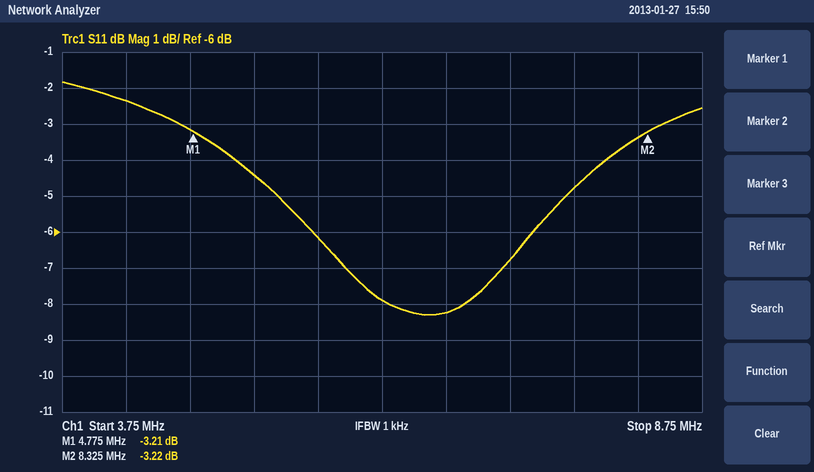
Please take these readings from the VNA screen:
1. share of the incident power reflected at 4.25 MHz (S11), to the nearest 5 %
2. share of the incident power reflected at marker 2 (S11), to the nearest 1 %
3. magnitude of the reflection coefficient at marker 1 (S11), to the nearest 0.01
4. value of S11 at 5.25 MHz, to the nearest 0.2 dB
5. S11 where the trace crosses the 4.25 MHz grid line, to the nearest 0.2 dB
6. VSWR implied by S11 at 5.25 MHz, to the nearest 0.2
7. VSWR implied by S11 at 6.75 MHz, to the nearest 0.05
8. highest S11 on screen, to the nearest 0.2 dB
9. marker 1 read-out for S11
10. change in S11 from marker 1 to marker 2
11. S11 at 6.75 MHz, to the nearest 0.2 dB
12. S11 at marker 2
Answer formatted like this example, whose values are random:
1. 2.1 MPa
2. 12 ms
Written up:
1. 60 %
2. 48 %
3. 0.69
4. -4.4 dB
5. -2.4 dB
6. 4.0
7. 2.25
8. -1.8 dB
9. -3.21 dB
10. -0.01 dB
11. -8.2 dB
12. -3.22 dB
